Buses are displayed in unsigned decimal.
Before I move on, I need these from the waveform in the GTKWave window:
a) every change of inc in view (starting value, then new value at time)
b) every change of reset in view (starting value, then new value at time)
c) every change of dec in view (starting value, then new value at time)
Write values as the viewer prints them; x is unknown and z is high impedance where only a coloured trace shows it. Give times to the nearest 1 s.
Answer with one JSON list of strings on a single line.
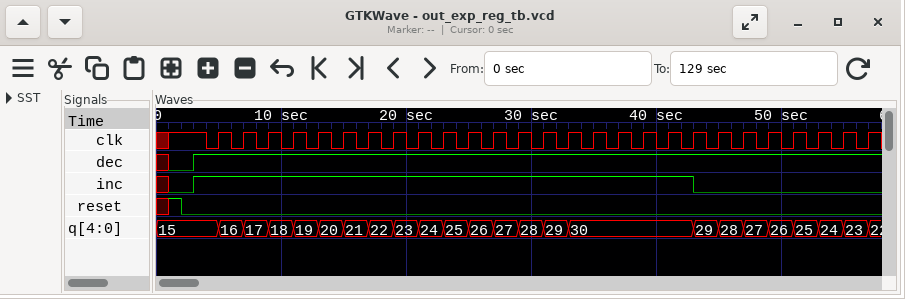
["x, 0 at 1 s, 1 at 3 s, 0 at 43 s", "x, 1 at 1 s, 0 at 2 s", "x, 0 at 1 s, 1 at 3 s"]
